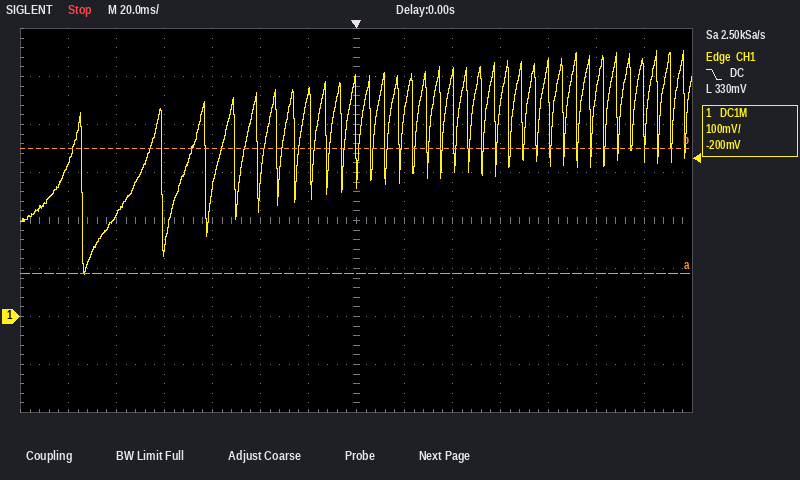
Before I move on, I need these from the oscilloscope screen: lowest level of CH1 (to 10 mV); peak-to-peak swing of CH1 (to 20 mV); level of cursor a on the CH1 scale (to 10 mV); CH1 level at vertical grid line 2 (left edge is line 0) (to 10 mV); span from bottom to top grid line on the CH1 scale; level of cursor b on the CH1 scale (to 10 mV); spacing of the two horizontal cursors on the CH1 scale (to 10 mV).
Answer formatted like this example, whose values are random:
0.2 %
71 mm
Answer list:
90 mV
460 mV
90 mV
210 mV
800 mV
350 mV
260 mV
